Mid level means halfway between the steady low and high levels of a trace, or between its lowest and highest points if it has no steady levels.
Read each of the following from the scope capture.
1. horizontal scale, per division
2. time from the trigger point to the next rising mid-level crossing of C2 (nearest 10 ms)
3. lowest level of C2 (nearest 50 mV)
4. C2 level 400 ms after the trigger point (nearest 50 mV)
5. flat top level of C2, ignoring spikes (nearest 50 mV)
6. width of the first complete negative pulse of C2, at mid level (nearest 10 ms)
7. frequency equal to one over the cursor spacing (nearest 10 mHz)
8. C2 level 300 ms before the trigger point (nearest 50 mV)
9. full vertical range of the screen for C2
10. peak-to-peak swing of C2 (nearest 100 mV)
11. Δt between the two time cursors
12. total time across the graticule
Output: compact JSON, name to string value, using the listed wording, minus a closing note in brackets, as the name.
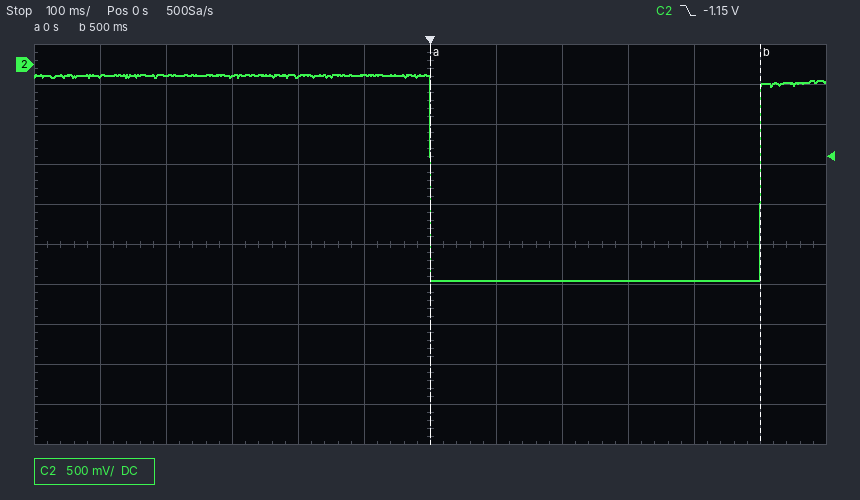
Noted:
{"horizontal scale, per division": "100 ms", "time from the trigger point to the next rising mid-level crossing of C2": "500 ms", "lowest level of C2": "-2.70 V", "C2 level 400 ms after the trigger point": "-2.70 V", "flat top level of C2, ignoring spikes": "-150 mV", "width of the first complete negative pulse of C2, at mid level": "500 ms", "frequency equal to one over the cursor spacing": "2.00 Hz", "C2 level 300 ms before the trigger point": "-150 mV", "full vertical range of the screen for C2": "5 V", "peak-to-peak swing of C2": "2.60 V", "Δt between the two time cursors": "500 ms", "total time across the graticule": "1.2 s"}
